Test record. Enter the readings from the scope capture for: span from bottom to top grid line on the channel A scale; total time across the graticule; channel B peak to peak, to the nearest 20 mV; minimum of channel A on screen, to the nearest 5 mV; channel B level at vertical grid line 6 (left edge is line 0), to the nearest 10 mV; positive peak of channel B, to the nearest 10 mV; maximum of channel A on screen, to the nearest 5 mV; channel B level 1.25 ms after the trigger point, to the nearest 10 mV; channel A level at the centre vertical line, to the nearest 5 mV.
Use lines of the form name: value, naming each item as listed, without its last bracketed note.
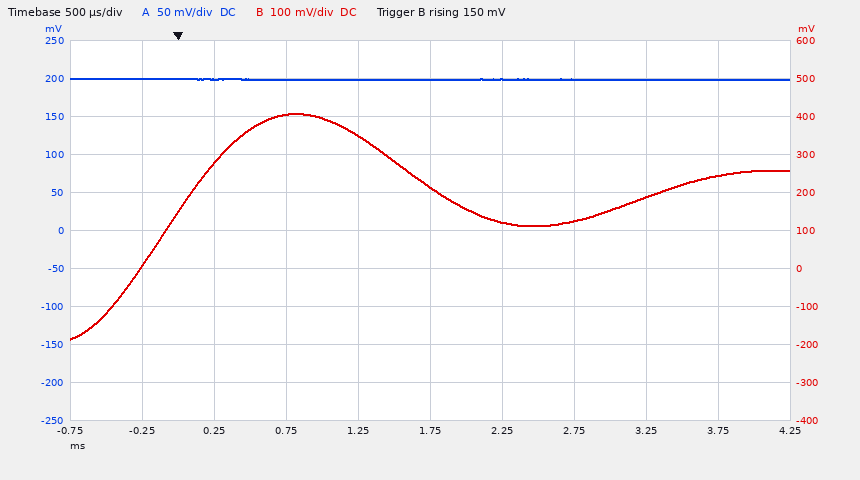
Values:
span from bottom to top grid line on the channel A scale: 500 mV
total time across the graticule: 5 ms
channel B peak to peak, to the nearest 20 mV: 600 mV
minimum of channel A on screen, to the nearest 5 mV: 200 mV
channel B level at vertical grid line 6 (left edge is line 0), to the nearest 10 mV: 120 mV
positive peak of channel B, to the nearest 10 mV: 410 mV
maximum of channel A on screen, to the nearest 5 mV: 200 mV
channel B level 1.25 ms after the trigger point, to the nearest 10 mV: 350 mV
channel A level at the centre vertical line, to the nearest 5 mV: 200 mV
